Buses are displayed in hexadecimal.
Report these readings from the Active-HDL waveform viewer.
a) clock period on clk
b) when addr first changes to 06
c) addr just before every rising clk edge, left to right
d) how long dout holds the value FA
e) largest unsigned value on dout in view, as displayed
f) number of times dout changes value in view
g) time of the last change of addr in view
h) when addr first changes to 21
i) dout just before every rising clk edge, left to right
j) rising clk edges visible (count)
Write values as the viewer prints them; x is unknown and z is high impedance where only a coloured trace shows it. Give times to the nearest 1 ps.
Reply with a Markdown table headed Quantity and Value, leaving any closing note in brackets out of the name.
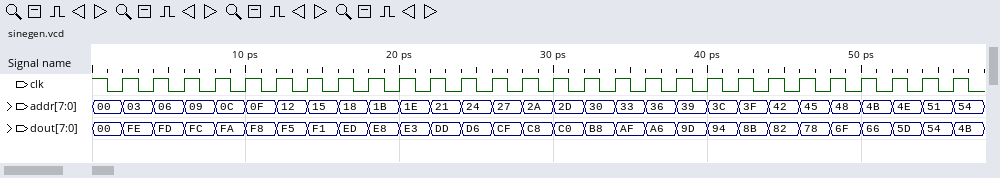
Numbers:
| Quantity | Value |
|---|---|
| clock period on clk | 2 ps |
| when addr first changes to 06 | 4 ps |
| addr just before every rising clk edge, left to right | 00, 03, 06, 09, 0C, 0F, 12, 15, 18, 1B, 1E, 21, 24, 27, 2A, 2D, 30, 33, 36, 39, 3C, 3F, 42, 45, 48, 4B, 4E, 51 |
| how long dout holds the value FA | 2 ps |
| largest unsigned value on dout in view, as displayed | FE |
| number of times dout changes value in view | 28 |
| time of the last change of addr in view | 56 ps |
| when addr first changes to 21 | 22 ps |
| dout just before every rising clk edge, left to right | 00, FE, FD, FC, FA, F8, F5, F1, ED, E8, E3, DD, D6, CF, C8, C0, B8, AF, A6, 9D, 94, 8B, 82, 78, 6F, 66, 5D, 54 |
| rising clk edges visible | 28 |
